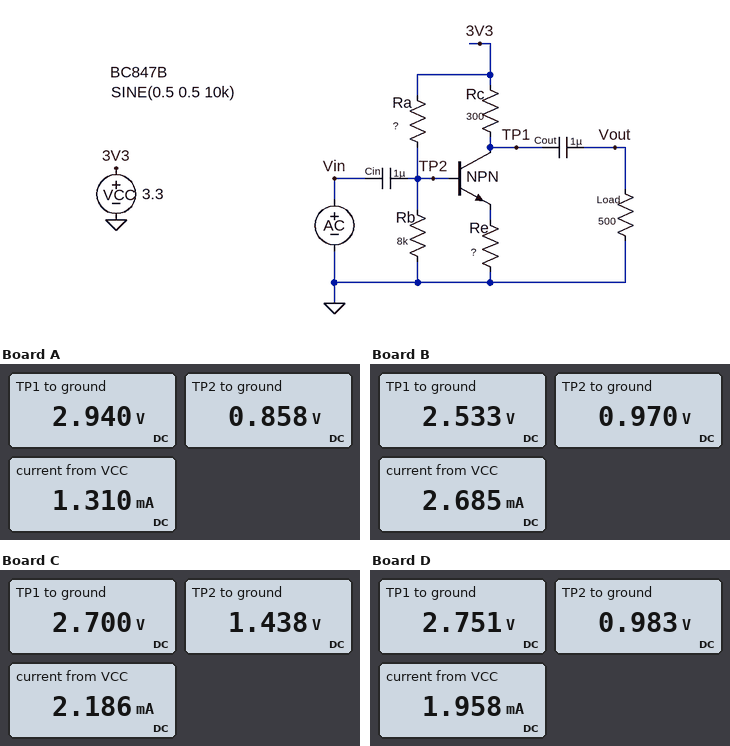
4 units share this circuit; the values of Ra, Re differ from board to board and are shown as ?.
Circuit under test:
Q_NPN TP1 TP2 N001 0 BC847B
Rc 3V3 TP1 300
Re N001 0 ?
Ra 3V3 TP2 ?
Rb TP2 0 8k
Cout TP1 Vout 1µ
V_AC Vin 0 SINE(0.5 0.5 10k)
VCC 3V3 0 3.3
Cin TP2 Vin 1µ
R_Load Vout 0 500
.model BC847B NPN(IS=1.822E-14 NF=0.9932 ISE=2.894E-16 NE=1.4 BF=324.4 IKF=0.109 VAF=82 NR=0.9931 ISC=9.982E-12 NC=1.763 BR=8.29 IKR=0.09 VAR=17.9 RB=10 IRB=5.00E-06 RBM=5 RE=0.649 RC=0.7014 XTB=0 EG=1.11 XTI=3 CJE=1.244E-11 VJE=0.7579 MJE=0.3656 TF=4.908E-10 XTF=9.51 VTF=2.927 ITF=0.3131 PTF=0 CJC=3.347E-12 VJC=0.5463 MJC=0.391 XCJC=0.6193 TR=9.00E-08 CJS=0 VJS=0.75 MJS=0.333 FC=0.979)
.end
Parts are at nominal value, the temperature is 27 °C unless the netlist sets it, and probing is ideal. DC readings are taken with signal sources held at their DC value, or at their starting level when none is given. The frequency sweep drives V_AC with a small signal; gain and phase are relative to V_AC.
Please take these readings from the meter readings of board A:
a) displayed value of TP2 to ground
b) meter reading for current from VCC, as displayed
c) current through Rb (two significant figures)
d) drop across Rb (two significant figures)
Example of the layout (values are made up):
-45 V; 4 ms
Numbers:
0.858 V; 1.310 mA; 110 µA; 860 mV
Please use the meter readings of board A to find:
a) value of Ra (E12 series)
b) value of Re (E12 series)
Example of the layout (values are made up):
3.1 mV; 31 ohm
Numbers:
22 kΩ; 180 Ω
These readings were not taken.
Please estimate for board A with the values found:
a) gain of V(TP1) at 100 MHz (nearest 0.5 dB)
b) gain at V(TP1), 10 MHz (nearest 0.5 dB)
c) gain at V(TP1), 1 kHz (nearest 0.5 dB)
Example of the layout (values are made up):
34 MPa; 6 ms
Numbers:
-1.0 dB; -0.5 dB; -0.5 dB
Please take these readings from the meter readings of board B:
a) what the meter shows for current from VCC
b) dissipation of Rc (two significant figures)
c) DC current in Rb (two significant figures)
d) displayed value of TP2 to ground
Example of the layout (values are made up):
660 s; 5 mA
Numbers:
2.685 mA; 2.0 mW; 120 µA; 0.970 V
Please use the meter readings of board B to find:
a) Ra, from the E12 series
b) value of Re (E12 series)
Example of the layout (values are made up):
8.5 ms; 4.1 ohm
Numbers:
18 kΩ; 120 Ω
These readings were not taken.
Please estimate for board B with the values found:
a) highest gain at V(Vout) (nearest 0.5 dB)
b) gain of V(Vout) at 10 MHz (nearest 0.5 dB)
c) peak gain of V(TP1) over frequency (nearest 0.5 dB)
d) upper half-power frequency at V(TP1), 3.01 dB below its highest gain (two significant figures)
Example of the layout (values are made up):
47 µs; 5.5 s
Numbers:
3.0 dB; 3.0 dB; 6.0 dB; 2.1 kHz
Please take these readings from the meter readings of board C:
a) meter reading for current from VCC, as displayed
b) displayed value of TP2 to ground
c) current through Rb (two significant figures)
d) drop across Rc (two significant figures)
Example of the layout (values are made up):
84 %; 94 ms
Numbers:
2.186 mA; 1.438 V; 180 µA; 600 mV
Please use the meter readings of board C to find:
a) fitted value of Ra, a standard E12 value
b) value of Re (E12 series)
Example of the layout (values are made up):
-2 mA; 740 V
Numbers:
10 kΩ; 390 Ω
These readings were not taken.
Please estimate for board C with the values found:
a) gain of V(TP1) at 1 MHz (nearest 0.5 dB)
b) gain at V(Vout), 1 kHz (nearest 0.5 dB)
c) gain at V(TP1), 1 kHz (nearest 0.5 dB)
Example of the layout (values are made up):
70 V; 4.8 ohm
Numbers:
-6.5 dB; -7.0 dB; -6.5 dB
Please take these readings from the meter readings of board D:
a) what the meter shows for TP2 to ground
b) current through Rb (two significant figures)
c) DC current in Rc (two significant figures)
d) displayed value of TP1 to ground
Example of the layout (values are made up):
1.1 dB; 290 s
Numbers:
0.983 V; 120 µA; 1.8 mA; 2.751 V
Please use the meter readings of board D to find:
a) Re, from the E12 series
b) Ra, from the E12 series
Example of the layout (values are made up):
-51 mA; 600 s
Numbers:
180 Ω; 18 kΩ
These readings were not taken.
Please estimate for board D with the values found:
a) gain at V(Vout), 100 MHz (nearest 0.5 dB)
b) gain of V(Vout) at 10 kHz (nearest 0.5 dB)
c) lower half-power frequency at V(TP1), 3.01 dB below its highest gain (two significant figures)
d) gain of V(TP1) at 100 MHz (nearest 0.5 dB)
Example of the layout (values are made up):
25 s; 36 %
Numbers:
-0.5 dB; -0.5 dB; 26 Hz; -0.5 dB
